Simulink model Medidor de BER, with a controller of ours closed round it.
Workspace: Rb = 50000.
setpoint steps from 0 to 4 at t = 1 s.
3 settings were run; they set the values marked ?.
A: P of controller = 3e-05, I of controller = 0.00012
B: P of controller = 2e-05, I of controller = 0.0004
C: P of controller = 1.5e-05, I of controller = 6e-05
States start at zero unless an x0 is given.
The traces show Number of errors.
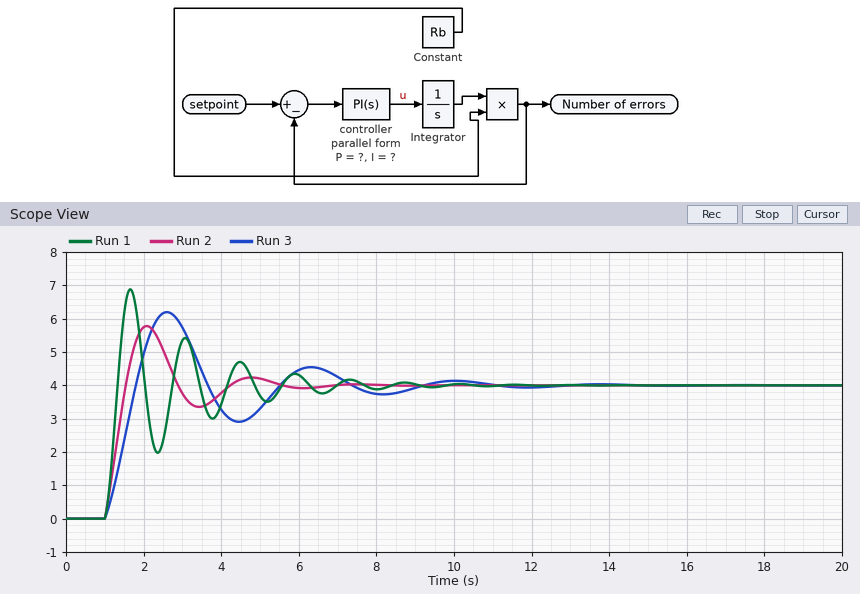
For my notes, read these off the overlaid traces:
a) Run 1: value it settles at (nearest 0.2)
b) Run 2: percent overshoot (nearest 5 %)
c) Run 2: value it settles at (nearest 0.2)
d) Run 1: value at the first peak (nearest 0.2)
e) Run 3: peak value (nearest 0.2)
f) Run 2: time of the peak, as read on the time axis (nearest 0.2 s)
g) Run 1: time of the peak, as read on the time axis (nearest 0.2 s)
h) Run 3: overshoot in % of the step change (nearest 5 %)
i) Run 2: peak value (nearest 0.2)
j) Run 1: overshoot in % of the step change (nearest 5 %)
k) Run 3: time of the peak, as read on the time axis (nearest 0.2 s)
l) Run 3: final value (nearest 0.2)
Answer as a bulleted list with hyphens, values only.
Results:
- 4.0
- 45 %
- 4.0
- 6.8
- 6.2
- 2.0 s
- 1.6 s
- 55 %
- 5.8
- 70 %
- 2.6 s
- 4.0
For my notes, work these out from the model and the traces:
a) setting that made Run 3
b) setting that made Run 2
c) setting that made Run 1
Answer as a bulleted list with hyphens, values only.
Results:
- C
- A
- B
